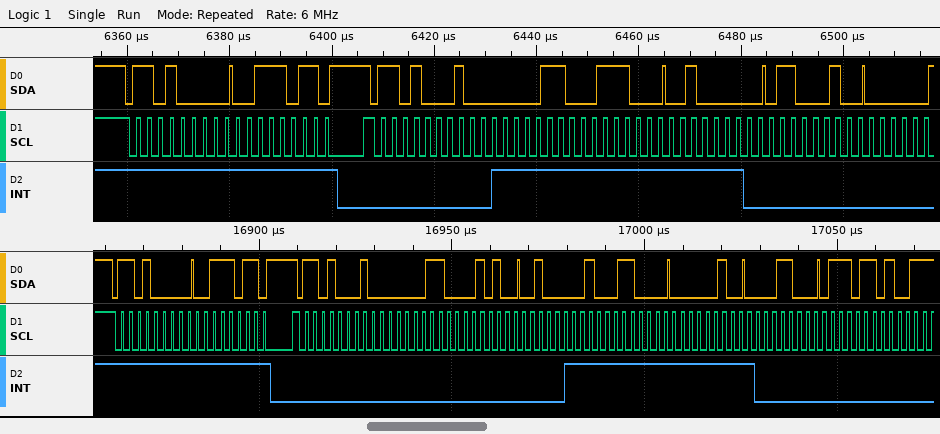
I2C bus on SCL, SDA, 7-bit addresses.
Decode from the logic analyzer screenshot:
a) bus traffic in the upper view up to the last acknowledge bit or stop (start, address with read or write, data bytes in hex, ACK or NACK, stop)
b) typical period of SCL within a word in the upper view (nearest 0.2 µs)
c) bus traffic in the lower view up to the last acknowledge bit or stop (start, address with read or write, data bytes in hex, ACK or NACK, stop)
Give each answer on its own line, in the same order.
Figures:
start, address 68 write ACK, 3B ACK, repeated start, address 68 read ACK, 03 ACK, 38 ACK, 40 ACK, C4 ACK
2.2 µs
start, address 68 write ACK, 3B ACK, repeated start, address 68 read ACK, 03 ACK, 14 ACK, 41 ACK, 30 ACK, 04 ACK, 18 ACK, ED ACK
